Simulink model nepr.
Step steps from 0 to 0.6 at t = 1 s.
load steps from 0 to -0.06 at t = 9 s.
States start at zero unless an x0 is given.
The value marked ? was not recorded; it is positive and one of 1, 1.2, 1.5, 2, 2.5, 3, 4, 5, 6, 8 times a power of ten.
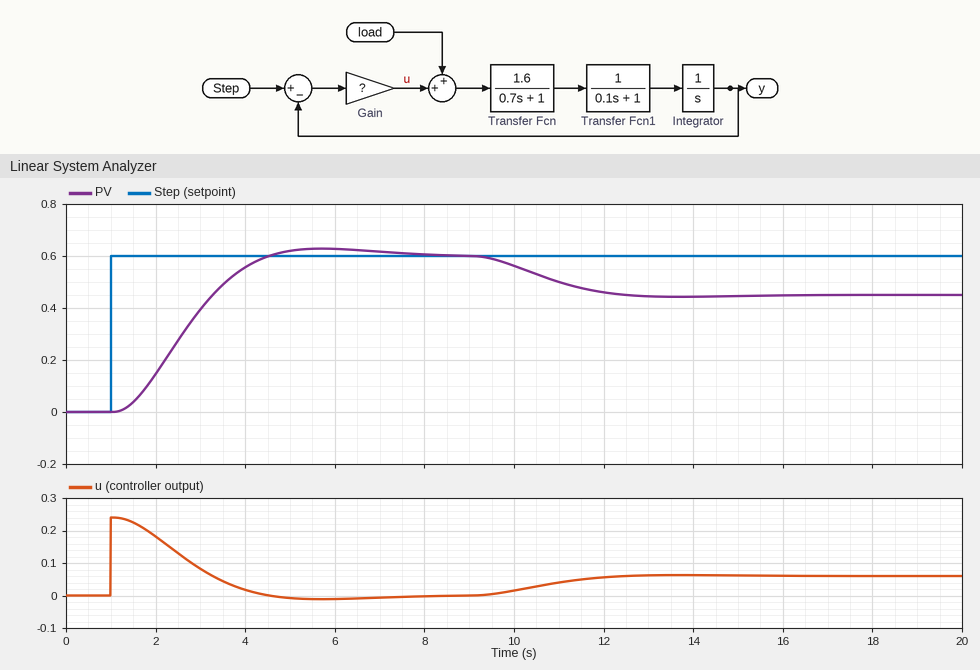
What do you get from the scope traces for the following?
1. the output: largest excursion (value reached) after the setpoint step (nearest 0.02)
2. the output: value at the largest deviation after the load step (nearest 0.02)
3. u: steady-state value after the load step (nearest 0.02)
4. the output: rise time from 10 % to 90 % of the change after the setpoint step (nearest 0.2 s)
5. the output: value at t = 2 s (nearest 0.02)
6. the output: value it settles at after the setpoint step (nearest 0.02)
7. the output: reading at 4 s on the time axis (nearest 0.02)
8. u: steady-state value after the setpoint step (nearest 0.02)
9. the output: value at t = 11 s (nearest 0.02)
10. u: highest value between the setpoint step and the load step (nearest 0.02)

0.62
0.44
0.06
2.2 s
0.14
0.60
0.56
0.00
0.50
0.24
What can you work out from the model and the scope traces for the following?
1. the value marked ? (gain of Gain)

0.4
